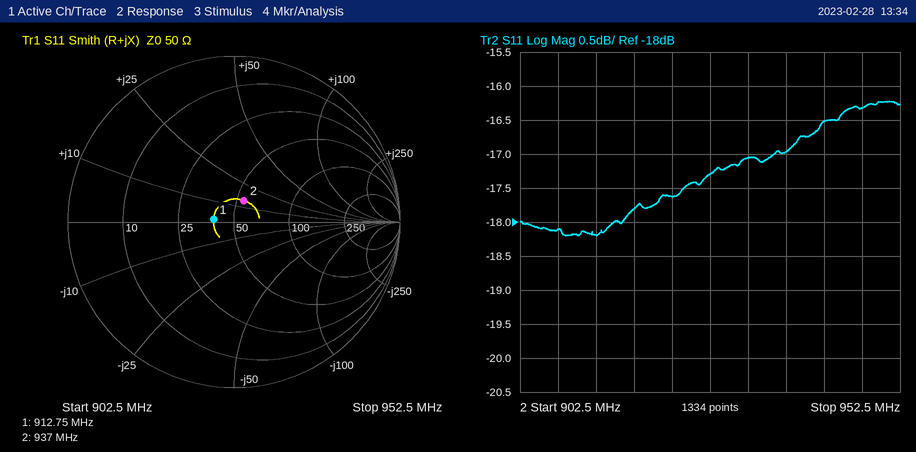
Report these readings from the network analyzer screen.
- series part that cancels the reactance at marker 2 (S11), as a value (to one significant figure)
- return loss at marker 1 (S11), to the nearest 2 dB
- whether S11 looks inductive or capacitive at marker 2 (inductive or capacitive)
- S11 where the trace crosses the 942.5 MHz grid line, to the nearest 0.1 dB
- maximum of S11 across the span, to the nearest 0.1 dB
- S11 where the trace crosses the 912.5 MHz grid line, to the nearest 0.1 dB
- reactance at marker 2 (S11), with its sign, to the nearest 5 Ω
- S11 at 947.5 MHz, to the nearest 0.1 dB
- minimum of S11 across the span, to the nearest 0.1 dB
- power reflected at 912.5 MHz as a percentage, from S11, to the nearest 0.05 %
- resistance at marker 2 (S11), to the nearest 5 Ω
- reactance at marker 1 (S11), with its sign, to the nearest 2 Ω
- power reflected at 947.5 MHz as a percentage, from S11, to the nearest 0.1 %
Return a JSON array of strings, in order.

["10 pF", "18 dB", "inductive", "-16.5 dB", "-16.2 dB", "-18.2 dB", "+15 Ω", "-16.3 dB", "-18.2 dB", "1.50 %", "55 Ω", "+2 Ω", "2.3 %"]
